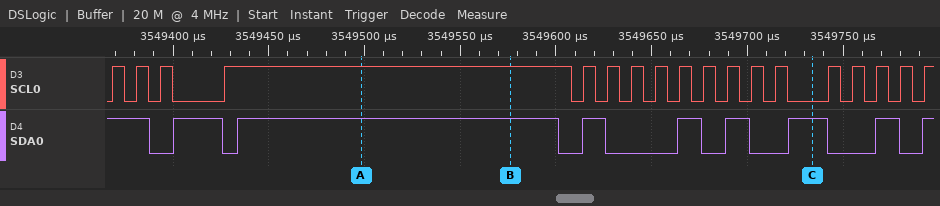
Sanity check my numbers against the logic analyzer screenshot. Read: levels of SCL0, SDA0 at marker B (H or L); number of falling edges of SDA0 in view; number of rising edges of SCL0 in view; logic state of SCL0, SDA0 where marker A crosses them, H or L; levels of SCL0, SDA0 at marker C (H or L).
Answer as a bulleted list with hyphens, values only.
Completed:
- SCL0=H, SDA0=H
- 8
- 18
- SCL0=H, SDA0=H
- SCL0=L, SDA0=H
